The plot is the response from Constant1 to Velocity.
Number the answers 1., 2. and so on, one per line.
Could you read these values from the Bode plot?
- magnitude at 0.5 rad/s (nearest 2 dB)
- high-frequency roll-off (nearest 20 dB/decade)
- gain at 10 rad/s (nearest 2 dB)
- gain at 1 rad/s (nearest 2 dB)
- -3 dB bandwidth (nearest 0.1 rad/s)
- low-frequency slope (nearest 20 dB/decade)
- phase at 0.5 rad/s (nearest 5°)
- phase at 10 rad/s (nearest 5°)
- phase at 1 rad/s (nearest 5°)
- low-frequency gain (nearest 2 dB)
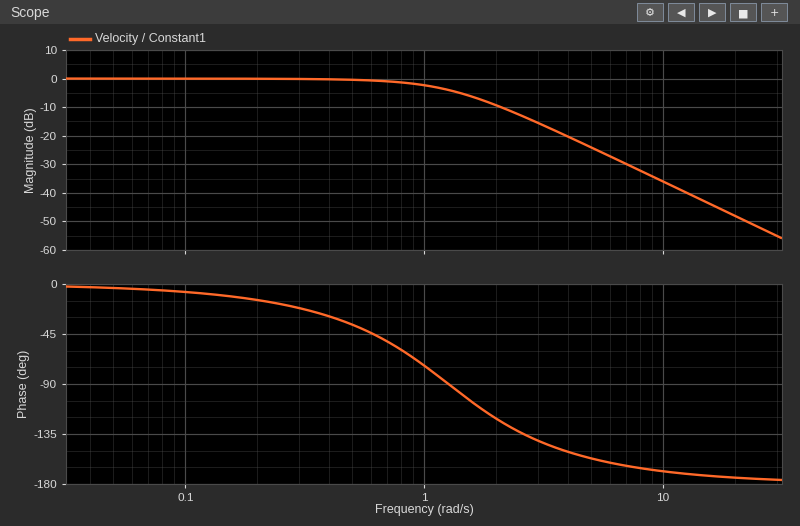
1. 0 dB
2. -40 dB/decade
3. -36 dB
4. -2 dB
5. 1.1 rad/s
6. 0 dB/decade
7. -35°
8. -170°
9. -75°
10. 0 dB
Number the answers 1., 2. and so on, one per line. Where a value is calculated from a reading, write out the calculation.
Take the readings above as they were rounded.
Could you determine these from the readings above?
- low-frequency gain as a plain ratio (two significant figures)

1. 10^(0 / 20) = 1.0
